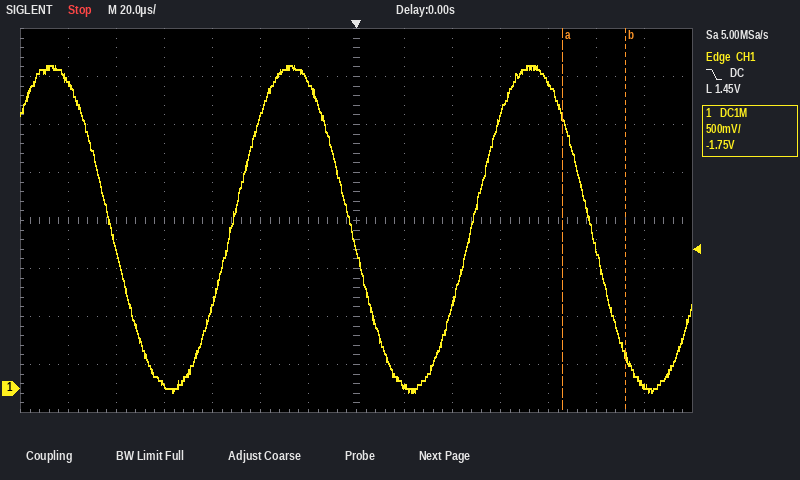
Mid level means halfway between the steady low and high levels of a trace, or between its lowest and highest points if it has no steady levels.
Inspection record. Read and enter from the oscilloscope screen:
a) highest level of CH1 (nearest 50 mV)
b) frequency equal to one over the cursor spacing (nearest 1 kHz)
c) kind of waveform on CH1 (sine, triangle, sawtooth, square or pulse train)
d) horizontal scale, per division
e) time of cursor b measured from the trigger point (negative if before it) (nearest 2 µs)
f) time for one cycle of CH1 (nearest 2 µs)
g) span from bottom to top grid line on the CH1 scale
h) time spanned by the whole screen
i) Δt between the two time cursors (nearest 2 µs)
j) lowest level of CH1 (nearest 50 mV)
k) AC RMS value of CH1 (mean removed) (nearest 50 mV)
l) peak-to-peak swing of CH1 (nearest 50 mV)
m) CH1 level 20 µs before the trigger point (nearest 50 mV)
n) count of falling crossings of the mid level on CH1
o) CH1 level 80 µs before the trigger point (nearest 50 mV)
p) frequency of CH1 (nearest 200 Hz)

3.35 V
38 kHz
sine
20 µs
+112 µs
100 µs
4 V
280 µs
26 µs
-50 mV
1.20 V
3.40 V
3.20 V
3
50 mV
10.0 kHz
